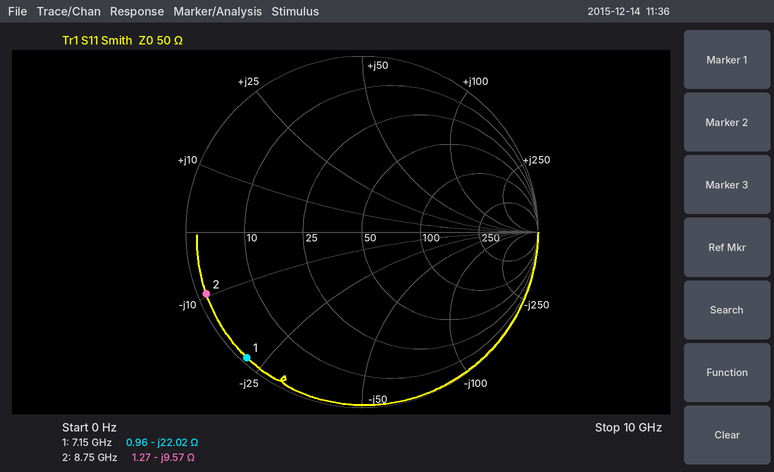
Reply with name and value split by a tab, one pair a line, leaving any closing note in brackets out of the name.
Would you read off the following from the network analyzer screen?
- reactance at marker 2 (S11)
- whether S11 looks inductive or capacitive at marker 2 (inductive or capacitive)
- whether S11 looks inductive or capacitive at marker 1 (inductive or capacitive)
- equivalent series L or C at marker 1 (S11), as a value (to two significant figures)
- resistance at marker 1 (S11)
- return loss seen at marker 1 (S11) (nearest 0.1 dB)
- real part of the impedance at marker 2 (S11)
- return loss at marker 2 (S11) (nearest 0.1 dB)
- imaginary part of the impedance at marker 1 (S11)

reactance at marker 2	-9.57 Ω
whether S11 looks inductive or capacitive at marker 2	capacitive
whether S11 looks inductive or capacitive at marker 1	capacitive
equivalent series L or C at marker 1 (S11), as a value	1.0 pF
resistance at marker 1	0.96 Ω
return loss seen at marker 1 (S11)	0.3 dB
real part of the impedance at marker 2	1.27 Ω
return loss at marker 2 (S11)	0.4 dB
imaginary part of the impedance at marker 1	-22.02 Ω
